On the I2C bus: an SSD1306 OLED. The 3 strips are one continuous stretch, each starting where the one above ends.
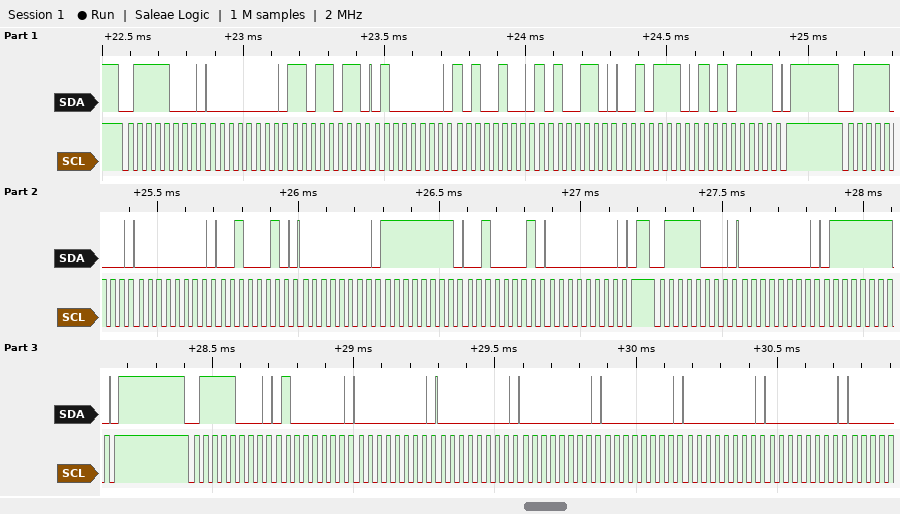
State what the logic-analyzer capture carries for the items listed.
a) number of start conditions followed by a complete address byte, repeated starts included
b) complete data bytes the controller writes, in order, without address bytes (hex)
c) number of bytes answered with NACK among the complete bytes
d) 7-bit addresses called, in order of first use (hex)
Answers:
4
00 DB 40 A4 A6 2E AF 00 22 00 FF 21 00 00 7F 40 00 00 00 00 00 00
0
0x3C
